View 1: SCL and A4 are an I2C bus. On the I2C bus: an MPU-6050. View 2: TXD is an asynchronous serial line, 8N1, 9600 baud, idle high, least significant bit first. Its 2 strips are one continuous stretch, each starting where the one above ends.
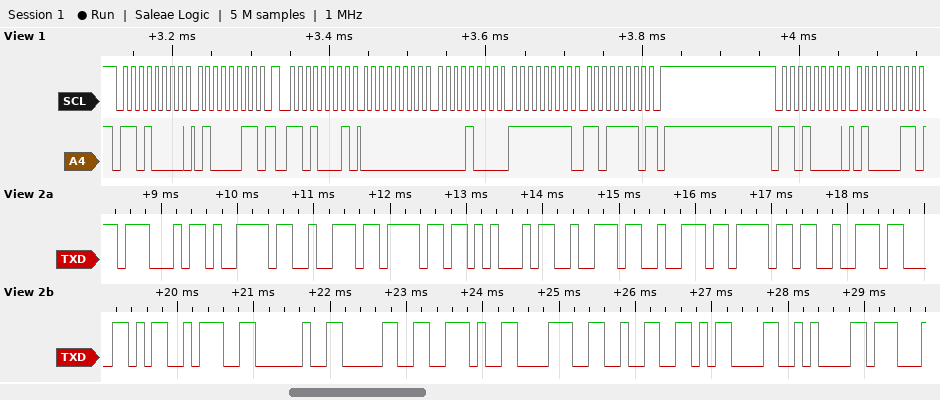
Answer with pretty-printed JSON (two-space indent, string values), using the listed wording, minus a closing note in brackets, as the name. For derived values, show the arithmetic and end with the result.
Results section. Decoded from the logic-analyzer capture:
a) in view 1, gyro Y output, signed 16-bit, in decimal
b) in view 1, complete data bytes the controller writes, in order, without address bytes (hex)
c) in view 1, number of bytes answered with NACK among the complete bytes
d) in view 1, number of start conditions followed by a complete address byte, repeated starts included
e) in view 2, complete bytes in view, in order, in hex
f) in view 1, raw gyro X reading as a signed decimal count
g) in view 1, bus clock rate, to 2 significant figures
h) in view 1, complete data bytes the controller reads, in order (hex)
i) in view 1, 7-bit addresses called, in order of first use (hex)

{
  "in view 1, gyro Y output, signed 16-bit, in decimal": "0xFFDE = -34",
  "in view 1, complete data bytes the controller writes, in order, without address bytes": "43 43",
  "in view 1, number of bytes answered with NACK among the complete bytes": "1",
  "in view 1, number of start conditions followed by a complete address byte, repeated starts included": "3",
  "in view 2, complete bytes in view, in order, in hex": "47 79 72 6F 45 72 72 6F 72 58 3A 20 30 2E 38 32 0D 0A",
  "in view 1, raw gyro X reading as a signed decimal count": "0x0008 = 8",
  "in view 1, bus clock rate, to 2 significant figures": "100 kHz",
  "in view 1, complete data bytes the controller reads, in order": "00 08 FF DE",
  "in view 1, 7-bit addresses called, in order of first use": "0x68"
}
